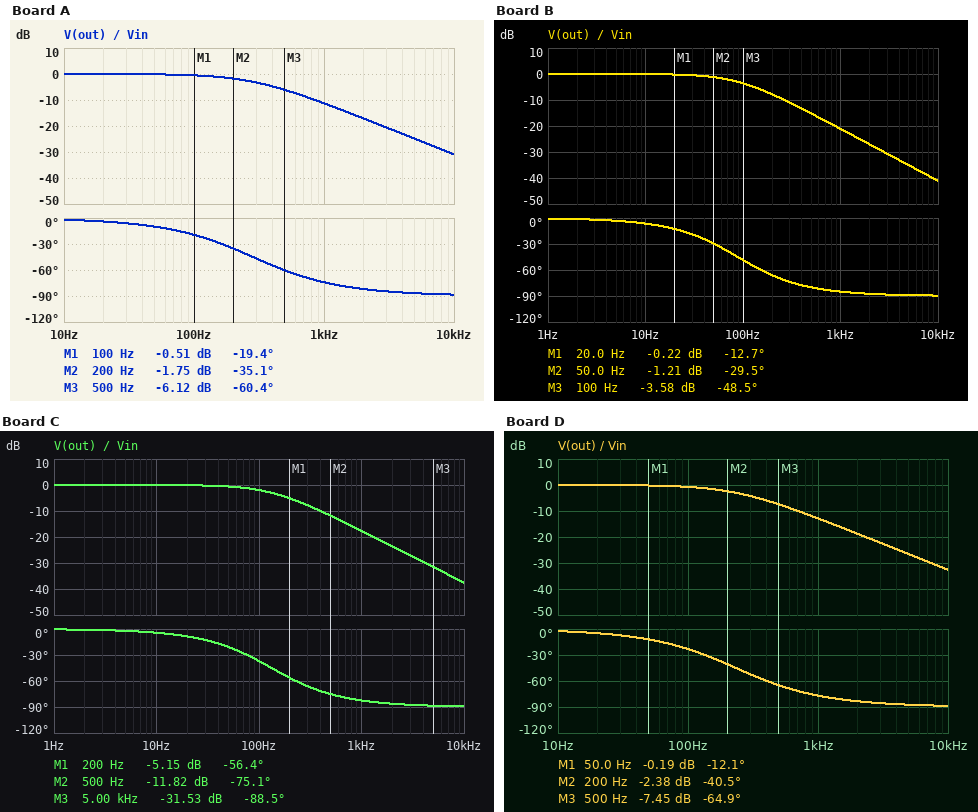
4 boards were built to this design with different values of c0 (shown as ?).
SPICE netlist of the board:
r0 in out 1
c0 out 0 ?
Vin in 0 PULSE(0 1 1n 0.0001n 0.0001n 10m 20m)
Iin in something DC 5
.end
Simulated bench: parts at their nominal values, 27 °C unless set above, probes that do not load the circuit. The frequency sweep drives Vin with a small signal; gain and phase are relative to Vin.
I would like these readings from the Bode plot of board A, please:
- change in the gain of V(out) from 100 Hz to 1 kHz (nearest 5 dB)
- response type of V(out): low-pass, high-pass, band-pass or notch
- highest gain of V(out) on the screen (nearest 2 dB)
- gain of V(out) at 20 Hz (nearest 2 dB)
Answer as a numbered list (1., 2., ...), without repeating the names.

1. -10 dB
2. low-pass
3. 0 dB
4. 0 dB
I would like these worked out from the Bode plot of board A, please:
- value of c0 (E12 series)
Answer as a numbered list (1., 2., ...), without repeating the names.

1. 560 µF
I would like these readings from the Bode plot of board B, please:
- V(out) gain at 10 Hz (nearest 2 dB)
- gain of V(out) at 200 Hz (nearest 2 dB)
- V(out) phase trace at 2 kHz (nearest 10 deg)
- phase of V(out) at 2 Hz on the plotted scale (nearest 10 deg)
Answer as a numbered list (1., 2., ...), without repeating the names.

1. 0 dB
2. -8 dB
3. -90 deg
4. 0 deg
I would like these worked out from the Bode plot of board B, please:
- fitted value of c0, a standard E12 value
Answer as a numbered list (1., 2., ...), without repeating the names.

1. 1.8 mF
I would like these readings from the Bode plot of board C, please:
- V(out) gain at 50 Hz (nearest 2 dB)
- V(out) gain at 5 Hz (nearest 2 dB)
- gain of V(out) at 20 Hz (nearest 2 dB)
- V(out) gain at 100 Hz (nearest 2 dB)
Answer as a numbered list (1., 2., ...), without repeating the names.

1. 0 dB
2. 0 dB
3. 0 dB
4. -2 dB
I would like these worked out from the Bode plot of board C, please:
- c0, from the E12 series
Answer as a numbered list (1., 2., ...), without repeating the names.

1. 1.2 mF
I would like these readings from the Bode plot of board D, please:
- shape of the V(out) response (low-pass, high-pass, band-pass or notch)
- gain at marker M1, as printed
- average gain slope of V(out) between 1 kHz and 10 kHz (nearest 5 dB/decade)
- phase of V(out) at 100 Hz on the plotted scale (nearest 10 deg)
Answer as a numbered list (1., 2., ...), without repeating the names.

1. low-pass
2. -0.19 dB
3. -20 dB/decade
4. -20 deg
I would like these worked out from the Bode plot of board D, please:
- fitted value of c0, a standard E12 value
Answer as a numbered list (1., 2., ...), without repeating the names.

1. 680 µF
